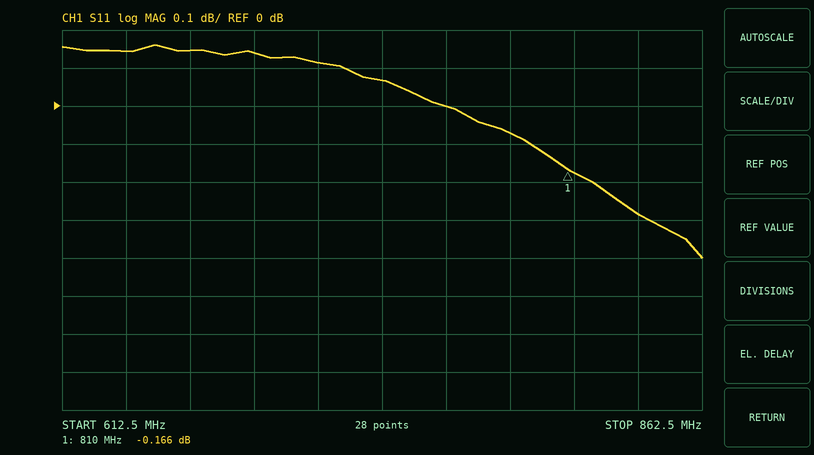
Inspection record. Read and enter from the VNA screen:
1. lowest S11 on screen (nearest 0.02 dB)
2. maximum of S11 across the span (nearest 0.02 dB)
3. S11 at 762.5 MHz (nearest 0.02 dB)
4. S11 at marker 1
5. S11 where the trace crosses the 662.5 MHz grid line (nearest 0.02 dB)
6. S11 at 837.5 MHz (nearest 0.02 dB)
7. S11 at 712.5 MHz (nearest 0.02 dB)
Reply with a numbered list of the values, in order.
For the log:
1. -0.40 dB
2. 0.16 dB
3. 0.00 dB
4. -0.166 dB
5. 0.14 dB
6. -0.28 dB
7. 0.12 dB
